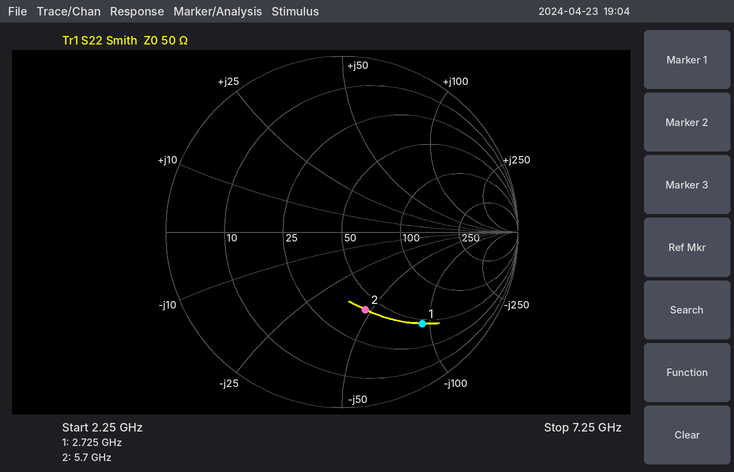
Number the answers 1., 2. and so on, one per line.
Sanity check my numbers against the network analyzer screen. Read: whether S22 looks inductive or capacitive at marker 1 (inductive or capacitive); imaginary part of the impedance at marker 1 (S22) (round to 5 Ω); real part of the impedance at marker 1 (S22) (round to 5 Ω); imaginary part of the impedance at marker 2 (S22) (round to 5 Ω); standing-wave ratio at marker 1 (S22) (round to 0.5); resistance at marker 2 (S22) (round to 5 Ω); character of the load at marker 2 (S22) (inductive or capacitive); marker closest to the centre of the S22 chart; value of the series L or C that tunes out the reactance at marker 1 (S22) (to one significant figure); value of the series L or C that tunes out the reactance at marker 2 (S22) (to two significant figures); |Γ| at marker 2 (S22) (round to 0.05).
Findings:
1. capacitive
2. -90 Ω
3. 45 Ω
4. -45 Ω
5. 5.5
6. 40 Ω
7. capacitive
8. marker 2
9. 5 nH
10. 1.3 nH
11. 0.45
